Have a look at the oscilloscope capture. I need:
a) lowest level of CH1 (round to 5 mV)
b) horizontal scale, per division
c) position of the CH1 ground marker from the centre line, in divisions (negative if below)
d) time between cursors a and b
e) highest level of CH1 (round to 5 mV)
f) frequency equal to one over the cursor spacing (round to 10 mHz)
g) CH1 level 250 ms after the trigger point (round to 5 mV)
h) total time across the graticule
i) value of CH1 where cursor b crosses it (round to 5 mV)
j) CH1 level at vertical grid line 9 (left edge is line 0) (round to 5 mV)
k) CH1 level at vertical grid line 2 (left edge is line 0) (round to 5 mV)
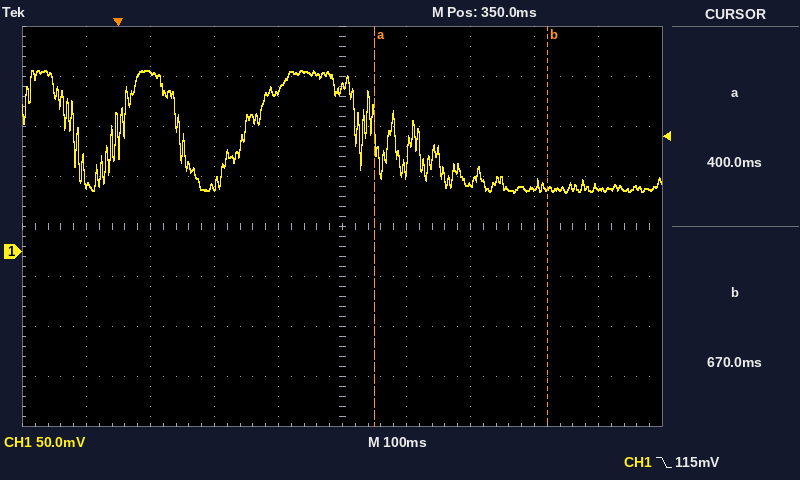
60 mV
100 ms
-0.5 div
270 ms
180 mV
3.70 Hz
160 mV
1 s
65 mV
65 mV
180 mV
